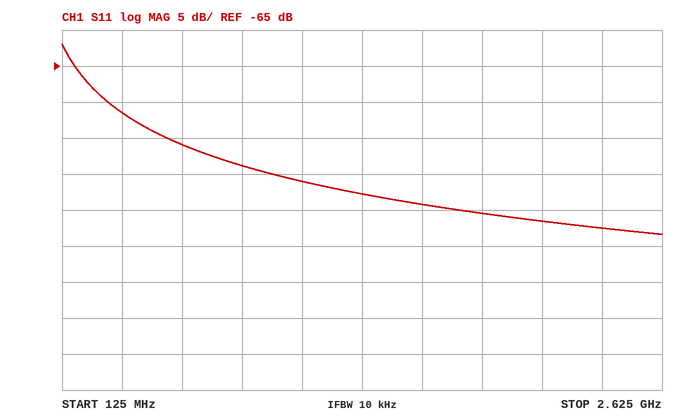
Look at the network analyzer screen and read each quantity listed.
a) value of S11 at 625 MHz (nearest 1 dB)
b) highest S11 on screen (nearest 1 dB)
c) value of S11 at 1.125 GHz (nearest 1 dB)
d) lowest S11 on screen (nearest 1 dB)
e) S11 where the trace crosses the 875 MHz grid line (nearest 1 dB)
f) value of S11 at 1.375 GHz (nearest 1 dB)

-76 dB
-62 dB
-81 dB
-88 dB
-79 dB
-83 dB
